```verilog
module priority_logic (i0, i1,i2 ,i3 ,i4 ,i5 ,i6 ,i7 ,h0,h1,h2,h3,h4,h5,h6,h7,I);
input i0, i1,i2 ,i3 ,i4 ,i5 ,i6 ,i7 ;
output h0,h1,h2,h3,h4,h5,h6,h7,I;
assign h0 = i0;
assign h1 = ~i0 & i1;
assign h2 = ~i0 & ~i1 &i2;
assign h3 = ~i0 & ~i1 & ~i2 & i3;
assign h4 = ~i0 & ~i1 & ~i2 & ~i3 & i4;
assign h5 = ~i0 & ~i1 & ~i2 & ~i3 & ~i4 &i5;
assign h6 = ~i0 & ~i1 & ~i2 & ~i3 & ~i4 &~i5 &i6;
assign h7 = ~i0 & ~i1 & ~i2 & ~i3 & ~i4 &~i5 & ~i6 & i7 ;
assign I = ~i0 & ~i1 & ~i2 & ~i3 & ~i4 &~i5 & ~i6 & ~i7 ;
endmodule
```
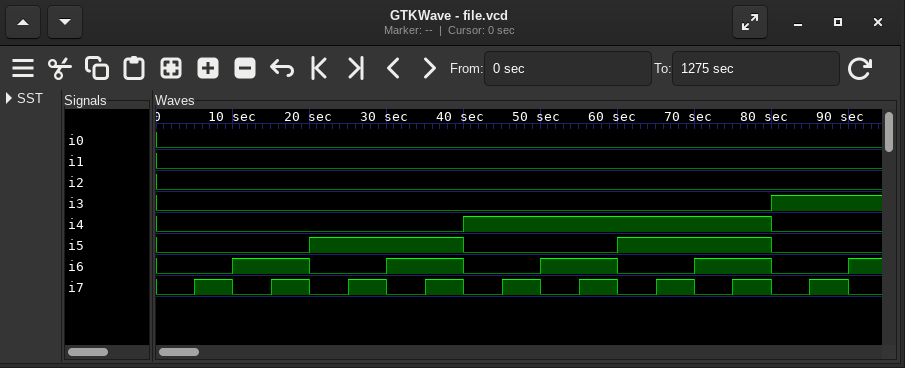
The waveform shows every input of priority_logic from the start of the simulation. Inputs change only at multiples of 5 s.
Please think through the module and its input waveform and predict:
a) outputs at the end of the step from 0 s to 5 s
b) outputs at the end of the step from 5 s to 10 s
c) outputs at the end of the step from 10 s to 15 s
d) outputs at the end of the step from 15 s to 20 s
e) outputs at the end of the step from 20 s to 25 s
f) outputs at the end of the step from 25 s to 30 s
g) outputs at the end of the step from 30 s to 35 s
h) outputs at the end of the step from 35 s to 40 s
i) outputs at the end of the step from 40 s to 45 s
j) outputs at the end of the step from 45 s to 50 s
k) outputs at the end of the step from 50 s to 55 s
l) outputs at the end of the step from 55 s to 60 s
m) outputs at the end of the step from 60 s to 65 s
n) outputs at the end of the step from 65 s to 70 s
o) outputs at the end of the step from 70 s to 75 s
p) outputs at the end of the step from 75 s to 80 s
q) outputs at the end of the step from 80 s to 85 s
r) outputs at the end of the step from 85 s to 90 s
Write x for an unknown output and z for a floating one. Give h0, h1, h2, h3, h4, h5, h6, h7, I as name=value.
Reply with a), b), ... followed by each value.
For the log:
a) h0=0, h1=0, h2=0, h3=0, h4=0, h5=0, h6=0, h7=0, I=1
b) h0=0, h1=0, h2=0, h3=0, h4=0, h5=0, h6=0, h7=1, I=0
c) h0=0, h1=0, h2=0, h3=0, h4=0, h5=0, h6=1, h7=0, I=0
d) h0=0, h1=0, h2=0, h3=0, h4=0, h5=0, h6=1, h7=0, I=0
e) h0=0, h1=0, h2=0, h3=0, h4=0, h5=1, h6=0, h7=0, I=0
f) h0=0, h1=0, h2=0, h3=0, h4=0, h5=1, h6=0, h7=0, I=0
g) h0=0, h1=0, h2=0, h3=0, h4=0, h5=1, h6=0, h7=0, I=0
h) h0=0, h1=0, h2=0, h3=0, h4=0, h5=1, h6=0, h7=0, I=0
i) h0=0, h1=0, h2=0, h3=0, h4=1, h5=0, h6=0, h7=0, I=0
j) h0=0, h1=0, h2=0, h3=0, h4=1, h5=0, h6=0, h7=0, I=0
k) h0=0, h1=0, h2=0, h3=0, h4=1, h5=0, h6=0, h7=0, I=0
l) h0=0, h1=0, h2=0, h3=0, h4=1, h5=0, h6=0, h7=0, I=0
m) h0=0, h1=0, h2=0, h3=0, h4=1, h5=0, h6=0, h7=0, I=0
n) h0=0, h1=0, h2=0, h3=0, h4=1, h5=0, h6=0, h7=0, I=0
o) h0=0, h1=0, h2=0, h3=0, h4=1, h5=0, h6=0, h7=0, I=0
p) h0=0, h1=0, h2=0, h3=0, h4=1, h5=0, h6=0, h7=0, I=0
q) h0=0, h1=0, h2=0, h3=1, h4=0, h5=0, h6=0, h7=0, I=0
r) h0=0, h1=0, h2=0, h3=1, h4=0, h5=0, h6=0, h7=0, I=0
